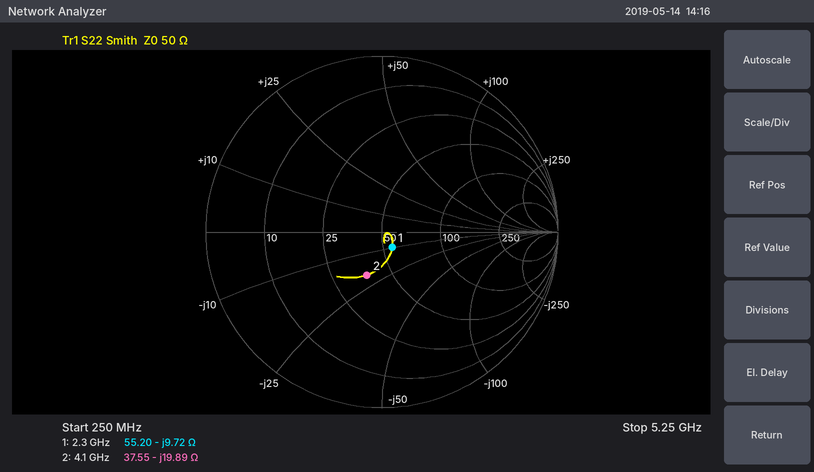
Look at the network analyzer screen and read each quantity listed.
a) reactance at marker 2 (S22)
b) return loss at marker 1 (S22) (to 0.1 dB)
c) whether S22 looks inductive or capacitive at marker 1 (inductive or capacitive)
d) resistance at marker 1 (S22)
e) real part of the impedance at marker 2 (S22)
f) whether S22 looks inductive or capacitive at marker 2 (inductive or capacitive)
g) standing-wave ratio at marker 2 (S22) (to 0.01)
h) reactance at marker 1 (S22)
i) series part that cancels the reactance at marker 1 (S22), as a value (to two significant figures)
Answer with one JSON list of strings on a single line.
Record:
["-19.89 Ω", "19.6 dB", "capacitive", "55.20 Ω", "37.55 Ω", "capacitive", "1.71", "-9.72 Ω", "670 pH"]
